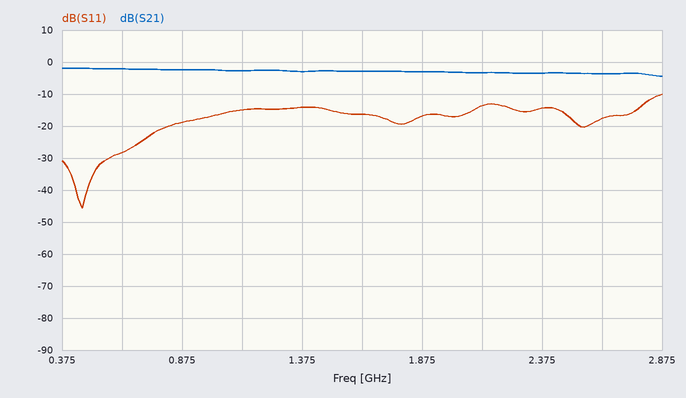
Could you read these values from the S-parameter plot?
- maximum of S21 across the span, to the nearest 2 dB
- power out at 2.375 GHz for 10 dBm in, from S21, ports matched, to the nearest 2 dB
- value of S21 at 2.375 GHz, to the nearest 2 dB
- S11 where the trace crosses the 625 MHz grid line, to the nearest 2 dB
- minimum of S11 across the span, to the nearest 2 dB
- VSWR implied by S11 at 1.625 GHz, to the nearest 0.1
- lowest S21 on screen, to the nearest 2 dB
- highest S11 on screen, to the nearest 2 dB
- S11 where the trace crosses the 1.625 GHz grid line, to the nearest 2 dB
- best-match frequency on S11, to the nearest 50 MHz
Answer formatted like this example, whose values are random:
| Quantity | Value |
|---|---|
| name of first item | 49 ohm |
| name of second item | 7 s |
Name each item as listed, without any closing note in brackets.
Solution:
| Quantity | Value |
|---|---|
| maximum of S21 across the span, to the nearest 2 dB | -2 dB |
| power out at 2.375 GHz for 10 dBm in, from S21, ports matched, to the nearest 2 dB | 6 dBm |
| value of S21 at 2.375 GHz, to the nearest 2 dB | -4 dB |
| S11 where the trace crosses the 625 MHz grid line, to the nearest 2 dB | -28 dB |
| minimum of S11 across the span, to the nearest 2 dB | -46 dB |
| VSWR implied by S11 at 1.625 GHz, to the nearest 0.1 | 1.4 |
| lowest S21 on screen, to the nearest 2 dB | -4 dB |
| highest S11 on screen, to the nearest 2 dB | -10 dB |
| S11 where the trace crosses the 1.625 GHz grid line, to the nearest 2 dB | -16 dB |
| best-match frequency on S11, to the nearest 50 MHz | 450 MHz |
